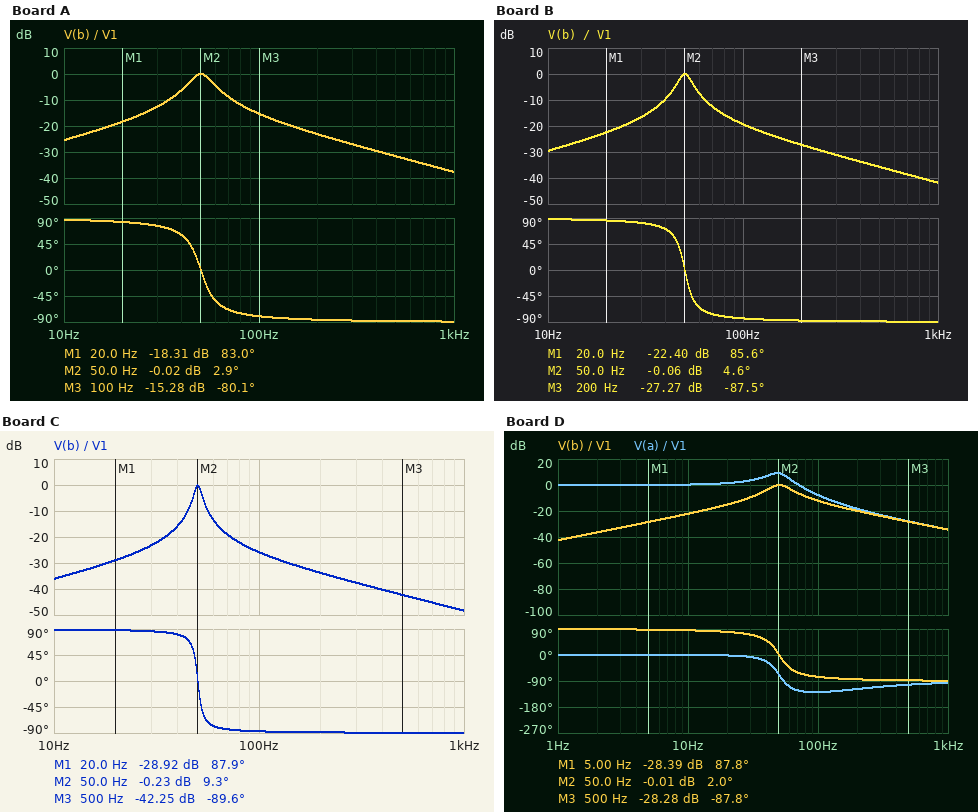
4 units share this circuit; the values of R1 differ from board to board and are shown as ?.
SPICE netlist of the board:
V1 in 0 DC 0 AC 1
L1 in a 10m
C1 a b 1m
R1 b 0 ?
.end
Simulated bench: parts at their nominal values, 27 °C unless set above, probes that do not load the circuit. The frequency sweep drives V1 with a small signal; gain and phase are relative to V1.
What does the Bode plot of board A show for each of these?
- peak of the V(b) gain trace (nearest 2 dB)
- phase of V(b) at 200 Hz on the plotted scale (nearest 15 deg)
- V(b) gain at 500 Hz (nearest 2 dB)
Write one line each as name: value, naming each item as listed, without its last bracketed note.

peak of the V(b) gain trace: 0 dB
phase of V(b) at 200 Hz on the plotted scale: -90 deg
V(b) gain at 500 Hz: -32 dB
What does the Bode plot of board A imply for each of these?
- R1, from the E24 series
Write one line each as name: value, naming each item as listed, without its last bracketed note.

R1, from the E24 series: 0.82 Ω
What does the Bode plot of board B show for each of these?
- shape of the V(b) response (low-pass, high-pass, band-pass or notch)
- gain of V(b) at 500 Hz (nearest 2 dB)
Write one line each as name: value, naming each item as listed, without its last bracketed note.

shape of the V(b) response: band-pass
gain of V(b) at 500 Hz: -36 dB
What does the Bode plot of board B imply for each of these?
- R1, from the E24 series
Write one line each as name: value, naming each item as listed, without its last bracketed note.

R1, from the E24 series: 0.51 Ω
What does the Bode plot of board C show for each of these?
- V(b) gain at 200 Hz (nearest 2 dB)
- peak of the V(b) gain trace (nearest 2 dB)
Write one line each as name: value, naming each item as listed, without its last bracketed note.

V(b) gain at 200 Hz: -34 dB
peak of the V(b) gain trace: 0 dB
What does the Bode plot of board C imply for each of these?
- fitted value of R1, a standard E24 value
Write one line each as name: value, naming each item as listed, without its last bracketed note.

fitted value of R1, a standard E24 value: 0.24 Ω
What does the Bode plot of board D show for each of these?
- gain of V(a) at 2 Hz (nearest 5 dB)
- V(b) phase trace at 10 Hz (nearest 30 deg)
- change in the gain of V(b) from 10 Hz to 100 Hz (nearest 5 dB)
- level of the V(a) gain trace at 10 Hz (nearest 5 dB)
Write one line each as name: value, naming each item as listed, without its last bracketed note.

gain of V(a) at 2 Hz: 0 dB
V(b) phase trace at 10 Hz: 90 deg
change in the gain of V(b) from 10 Hz to 100 Hz: 10 dB
level of the V(a) gain trace at 10 Hz: 0 dB
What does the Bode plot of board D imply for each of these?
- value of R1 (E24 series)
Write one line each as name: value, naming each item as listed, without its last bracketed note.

value of R1: 1.2 Ω
